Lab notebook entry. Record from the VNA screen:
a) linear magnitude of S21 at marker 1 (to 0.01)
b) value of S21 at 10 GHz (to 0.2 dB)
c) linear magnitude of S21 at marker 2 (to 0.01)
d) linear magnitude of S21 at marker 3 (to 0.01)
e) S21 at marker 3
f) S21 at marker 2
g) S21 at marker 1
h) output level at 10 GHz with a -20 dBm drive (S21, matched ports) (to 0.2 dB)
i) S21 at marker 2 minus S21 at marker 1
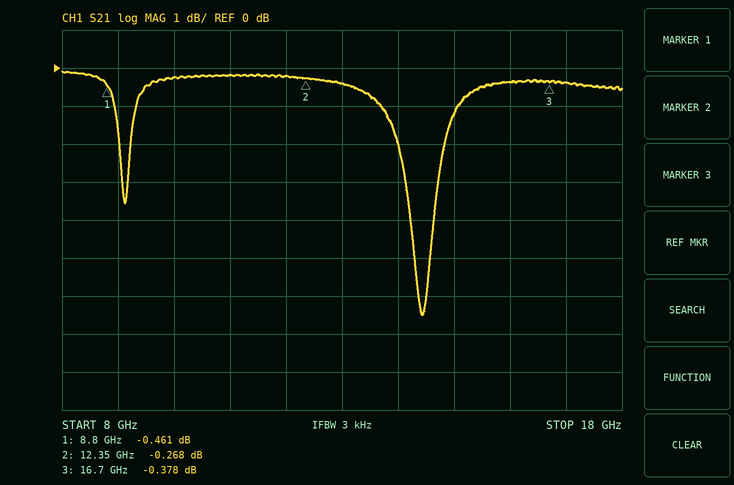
0.95
-0.2 dB
0.97
0.96
-0.378 dB
-0.268 dB
-0.461 dB
-20.2 dBm
0.193 dB
